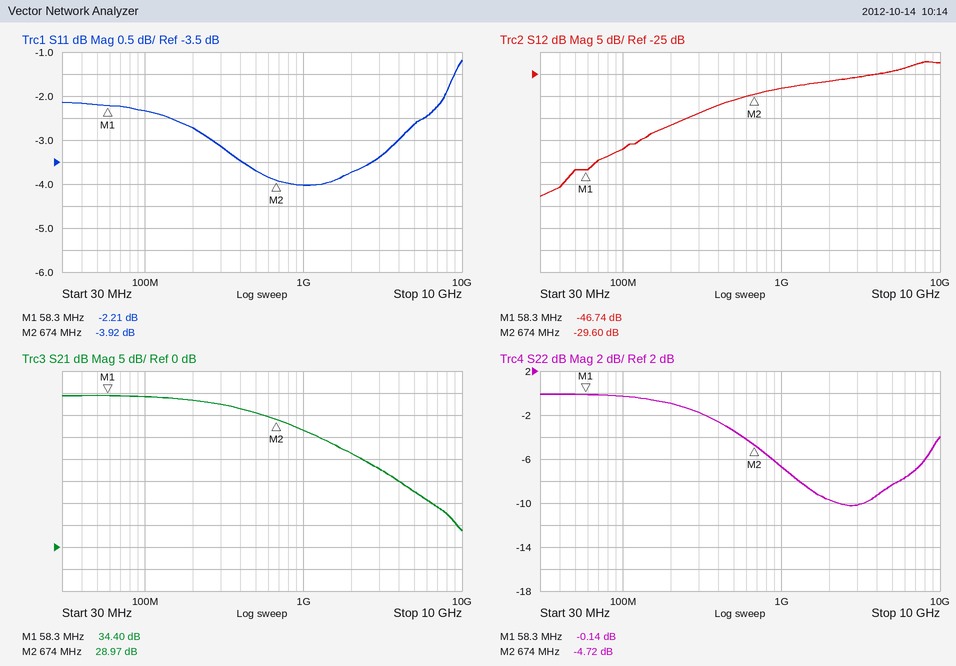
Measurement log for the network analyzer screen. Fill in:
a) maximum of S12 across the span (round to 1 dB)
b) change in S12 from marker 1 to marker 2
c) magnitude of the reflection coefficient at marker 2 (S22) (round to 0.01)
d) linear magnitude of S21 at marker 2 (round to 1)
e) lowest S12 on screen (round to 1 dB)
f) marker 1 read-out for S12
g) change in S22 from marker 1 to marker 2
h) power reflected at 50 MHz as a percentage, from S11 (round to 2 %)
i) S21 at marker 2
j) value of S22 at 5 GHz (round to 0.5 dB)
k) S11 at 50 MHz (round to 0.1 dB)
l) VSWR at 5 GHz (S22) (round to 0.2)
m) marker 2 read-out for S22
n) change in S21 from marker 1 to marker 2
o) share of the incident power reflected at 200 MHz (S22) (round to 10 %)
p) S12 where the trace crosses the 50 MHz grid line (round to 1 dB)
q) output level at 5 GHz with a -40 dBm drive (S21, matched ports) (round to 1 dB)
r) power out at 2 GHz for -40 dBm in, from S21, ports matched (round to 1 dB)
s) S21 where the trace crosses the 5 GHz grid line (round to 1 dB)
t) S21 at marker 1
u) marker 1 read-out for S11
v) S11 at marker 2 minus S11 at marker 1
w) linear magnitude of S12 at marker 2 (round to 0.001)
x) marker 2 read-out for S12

-22 dB
17.14 dB
0.58
28
-53 dB
-46.74 dB
-4.58 dB
60 %
28.97 dB
-8.5 dB
-2.2 dB
2.2
-4.72 dB
-5.43 dB
80 %
-47 dB
-27 dBm
-19 dBm
13 dB
34.40 dB
-2.21 dB
-1.71 dB
0.033
-29.60 dB
